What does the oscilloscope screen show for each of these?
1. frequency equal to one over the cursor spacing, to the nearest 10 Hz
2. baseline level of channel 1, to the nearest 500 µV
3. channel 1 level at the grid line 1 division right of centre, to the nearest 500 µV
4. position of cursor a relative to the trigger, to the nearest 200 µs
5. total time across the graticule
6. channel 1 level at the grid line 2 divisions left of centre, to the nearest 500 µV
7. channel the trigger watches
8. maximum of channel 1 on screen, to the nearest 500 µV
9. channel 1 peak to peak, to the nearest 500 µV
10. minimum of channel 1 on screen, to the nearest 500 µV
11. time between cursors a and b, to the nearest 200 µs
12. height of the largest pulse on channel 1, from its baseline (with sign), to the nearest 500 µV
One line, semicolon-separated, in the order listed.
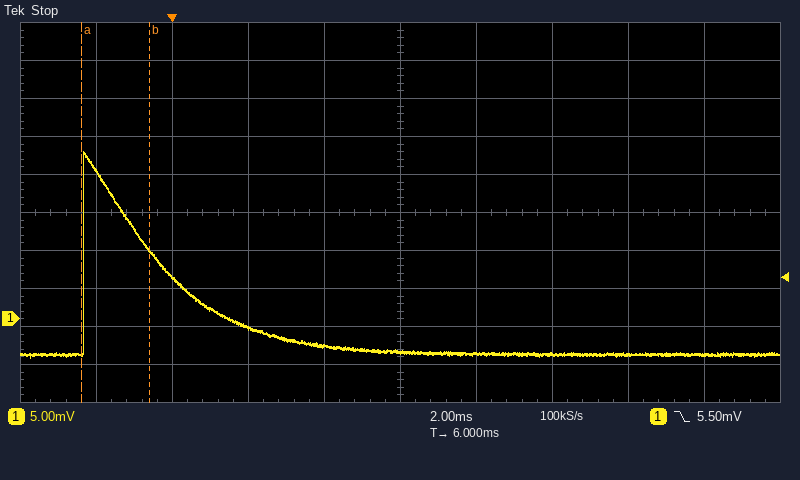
560 Hz; -4.5 mV; -4.5 mV; -2.4 ms; 20 ms; -1.0 mV; channel 1; 22.0 mV; 27.0 mV; -5.0 mV; 1.8 ms; +26.5 mV
